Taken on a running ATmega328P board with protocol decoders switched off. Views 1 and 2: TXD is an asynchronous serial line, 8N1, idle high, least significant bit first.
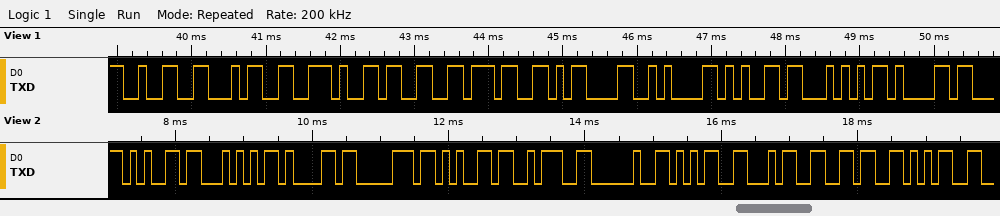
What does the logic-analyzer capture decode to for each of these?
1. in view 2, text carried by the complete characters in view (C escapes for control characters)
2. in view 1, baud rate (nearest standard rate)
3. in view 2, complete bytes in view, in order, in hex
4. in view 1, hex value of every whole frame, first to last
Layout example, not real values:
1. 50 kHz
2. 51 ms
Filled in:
1. "eTape: 5465"
2. 9600 baud
3. 65 54 61 70 65 3A 20 35 34 36 35
4. 32 34 2E 33 37 0D 0A 65 54 61
